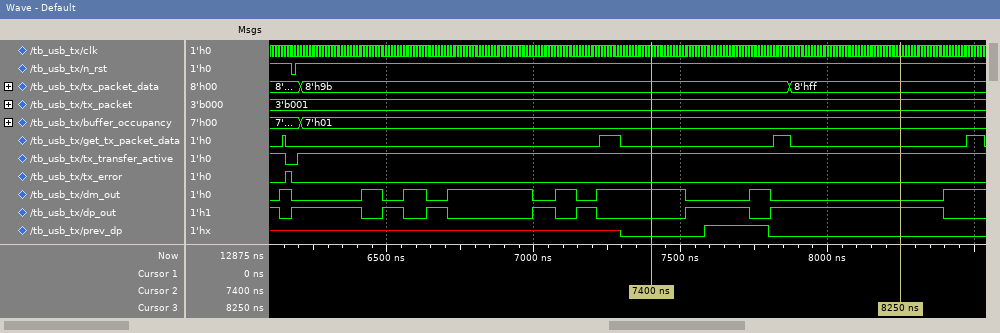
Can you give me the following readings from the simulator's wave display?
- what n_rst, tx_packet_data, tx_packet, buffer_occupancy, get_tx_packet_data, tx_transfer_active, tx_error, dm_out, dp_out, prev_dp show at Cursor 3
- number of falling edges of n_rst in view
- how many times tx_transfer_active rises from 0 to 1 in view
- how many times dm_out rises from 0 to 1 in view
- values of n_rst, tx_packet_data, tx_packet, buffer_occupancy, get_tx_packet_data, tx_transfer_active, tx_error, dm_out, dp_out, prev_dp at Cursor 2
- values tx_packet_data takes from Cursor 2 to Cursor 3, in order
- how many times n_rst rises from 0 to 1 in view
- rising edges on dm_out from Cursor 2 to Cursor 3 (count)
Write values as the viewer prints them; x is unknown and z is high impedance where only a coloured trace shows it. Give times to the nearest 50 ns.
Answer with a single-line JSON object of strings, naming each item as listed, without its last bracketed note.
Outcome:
{"what n_rst, tx_packet_data, tx_packet, buffer_occupancy, get_tx_packet_data, tx_transfer_active, tx_error, dm_out, dp_out, prev_dp show at Cursor 3": "n_rst=1, tx_packet_data=8'hff, tx_packet=3'b001, buffer_occupancy=7'h01, get_tx_packet_data=0, tx_transfer_active=1, tx_error=0, dm_out=0, dp_out=1, prev_dp=0", "number of falling edges of n_rst in view": "1", "how many times tx_transfer_active rises from 0 to 1 in view": "1", "how many times dm_out rises from 0 to 1 in view": "8", "values of n_rst, tx_packet_data, tx_packet, buffer_occupancy, get_tx_packet_data, tx_transfer_active, tx_error, dm_out, dp_out, prev_dp at Cursor 2": "n_rst=1, tx_packet_data=8'h9b, tx_packet=3'b001, buffer_occupancy=7'h01, get_tx_packet_data=0, tx_transfer_active=1, tx_error=0, dm_out=1, dp_out=0, prev_dp=0", "values tx_packet_data takes from Cursor 2 to Cursor 3, in order": "8'h9b, 8'hff", "how many times n_rst rises from 0 to 1 in view": "1", "rising edges on dm_out from Cursor 2 to Cursor 3": "1"}
